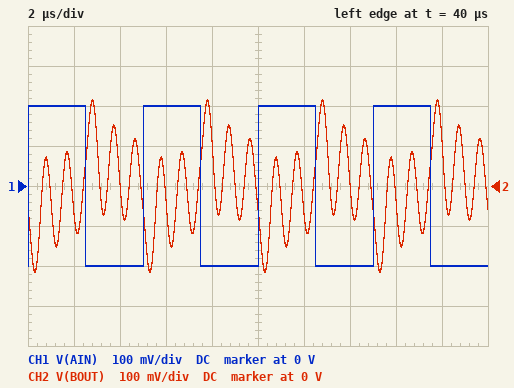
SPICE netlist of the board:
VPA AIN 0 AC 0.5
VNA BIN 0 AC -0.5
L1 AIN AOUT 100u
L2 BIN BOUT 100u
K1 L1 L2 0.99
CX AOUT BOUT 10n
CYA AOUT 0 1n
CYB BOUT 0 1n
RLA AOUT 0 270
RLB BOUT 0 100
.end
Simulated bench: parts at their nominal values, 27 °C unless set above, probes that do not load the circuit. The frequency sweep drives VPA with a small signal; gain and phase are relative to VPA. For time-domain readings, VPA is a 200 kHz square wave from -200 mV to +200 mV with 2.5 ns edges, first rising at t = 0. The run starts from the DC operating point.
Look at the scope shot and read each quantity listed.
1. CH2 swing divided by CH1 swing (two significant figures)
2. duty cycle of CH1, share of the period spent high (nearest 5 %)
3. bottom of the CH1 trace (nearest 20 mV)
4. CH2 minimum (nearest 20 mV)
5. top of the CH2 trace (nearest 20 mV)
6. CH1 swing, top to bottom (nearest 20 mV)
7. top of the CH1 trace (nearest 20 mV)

1.1
50 %
-200 mV
-220 mV
220 mV
400 mV
200 mV
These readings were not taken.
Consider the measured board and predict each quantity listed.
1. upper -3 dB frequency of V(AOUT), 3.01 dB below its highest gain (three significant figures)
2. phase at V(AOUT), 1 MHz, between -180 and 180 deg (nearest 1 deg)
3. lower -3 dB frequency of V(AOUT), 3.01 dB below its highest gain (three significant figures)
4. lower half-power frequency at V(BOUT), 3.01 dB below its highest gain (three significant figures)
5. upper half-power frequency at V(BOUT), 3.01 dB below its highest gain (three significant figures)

1.12 MHz
-23 deg
1.07 MHz
1.07 MHz
1.12 MHz
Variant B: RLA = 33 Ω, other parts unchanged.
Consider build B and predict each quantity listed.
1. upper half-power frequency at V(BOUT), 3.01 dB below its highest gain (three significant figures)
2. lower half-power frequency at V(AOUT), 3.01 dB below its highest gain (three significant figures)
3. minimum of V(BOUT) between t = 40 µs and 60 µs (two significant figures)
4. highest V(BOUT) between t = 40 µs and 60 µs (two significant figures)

1.15 MHz
1.03 MHz
-430 mV
430 mV
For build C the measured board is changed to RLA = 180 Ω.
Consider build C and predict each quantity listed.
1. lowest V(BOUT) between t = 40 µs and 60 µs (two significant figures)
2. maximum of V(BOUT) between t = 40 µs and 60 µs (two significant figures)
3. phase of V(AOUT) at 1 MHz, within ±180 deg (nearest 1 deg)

-240 mV
240 mV
-22 deg
